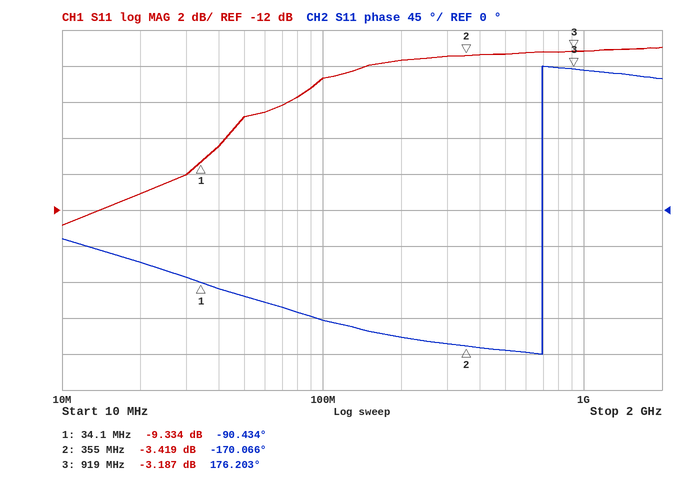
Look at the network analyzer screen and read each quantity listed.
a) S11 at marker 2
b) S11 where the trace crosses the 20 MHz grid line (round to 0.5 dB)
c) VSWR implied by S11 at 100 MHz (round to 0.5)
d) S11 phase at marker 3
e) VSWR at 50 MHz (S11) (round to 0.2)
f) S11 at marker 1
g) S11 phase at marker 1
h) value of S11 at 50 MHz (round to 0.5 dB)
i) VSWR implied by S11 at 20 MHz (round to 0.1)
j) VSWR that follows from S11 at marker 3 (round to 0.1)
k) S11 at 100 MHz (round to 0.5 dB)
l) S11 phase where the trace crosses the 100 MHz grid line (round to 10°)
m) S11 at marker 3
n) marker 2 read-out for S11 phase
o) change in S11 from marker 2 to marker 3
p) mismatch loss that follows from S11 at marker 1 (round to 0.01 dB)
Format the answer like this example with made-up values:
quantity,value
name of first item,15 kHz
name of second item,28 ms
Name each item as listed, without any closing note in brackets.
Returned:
quantity,value
S11 at marker 2,-3.419 dB
S11 where the trace crosses the 20 MHz grid line,-11.0 dB
VSWR implied by S11 at 100 MHz,4.0
S11 phase at marker 3,176.203°
VSWR at 50 MHz (S11),2.6
S11 at marker 1,-9.334 dB
S11 phase at marker 1,-90.434°
value of S11 at 50 MHz,-7.0 dB
VSWR implied by S11 at 20 MHz,1.8
VSWR that follows from S11 at marker 3,5.5
S11 at 100 MHz,-4.5 dB
S11 phase where the trace crosses the 100 MHz grid line,-140°
S11 at marker 3,-3.187 dB
marker 2 read-out for S11 phase,-170.066°
change in S11 from marker 2 to marker 3,0.232 dB
mismatch loss that follows from S11 at marker 1,0.54 dB
